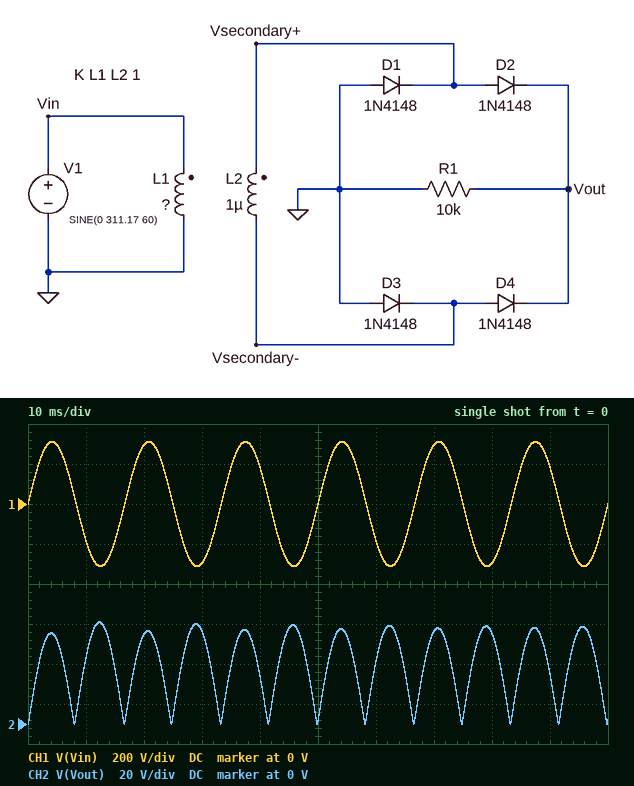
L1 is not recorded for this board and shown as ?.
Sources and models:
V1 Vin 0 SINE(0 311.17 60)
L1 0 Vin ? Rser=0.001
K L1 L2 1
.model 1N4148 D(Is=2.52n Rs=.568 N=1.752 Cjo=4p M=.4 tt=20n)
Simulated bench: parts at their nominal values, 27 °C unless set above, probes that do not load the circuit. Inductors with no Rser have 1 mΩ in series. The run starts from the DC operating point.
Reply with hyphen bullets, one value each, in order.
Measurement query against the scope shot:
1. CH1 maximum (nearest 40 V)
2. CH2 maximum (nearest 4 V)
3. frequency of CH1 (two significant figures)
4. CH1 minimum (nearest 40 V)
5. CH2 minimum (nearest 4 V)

- 320 V
- 52 V
- 60 Hz
- -320 V
- 0 V
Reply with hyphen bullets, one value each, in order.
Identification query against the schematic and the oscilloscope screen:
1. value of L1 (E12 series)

- 39 µH
